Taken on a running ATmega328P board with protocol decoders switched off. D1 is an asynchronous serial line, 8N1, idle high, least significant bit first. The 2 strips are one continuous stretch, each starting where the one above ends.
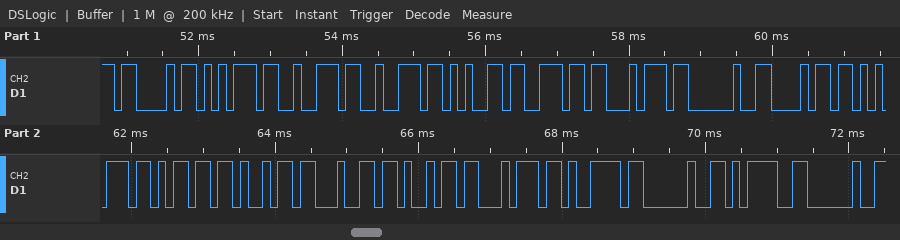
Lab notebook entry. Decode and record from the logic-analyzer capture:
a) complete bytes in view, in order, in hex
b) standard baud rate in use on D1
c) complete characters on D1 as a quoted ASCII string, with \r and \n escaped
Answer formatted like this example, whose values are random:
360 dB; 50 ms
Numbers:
43 75 72 72 65 6E 74 20 68 75 6D 69 64 69 74 79 20 3D 20; 9600 baud; "Current humidity = "
